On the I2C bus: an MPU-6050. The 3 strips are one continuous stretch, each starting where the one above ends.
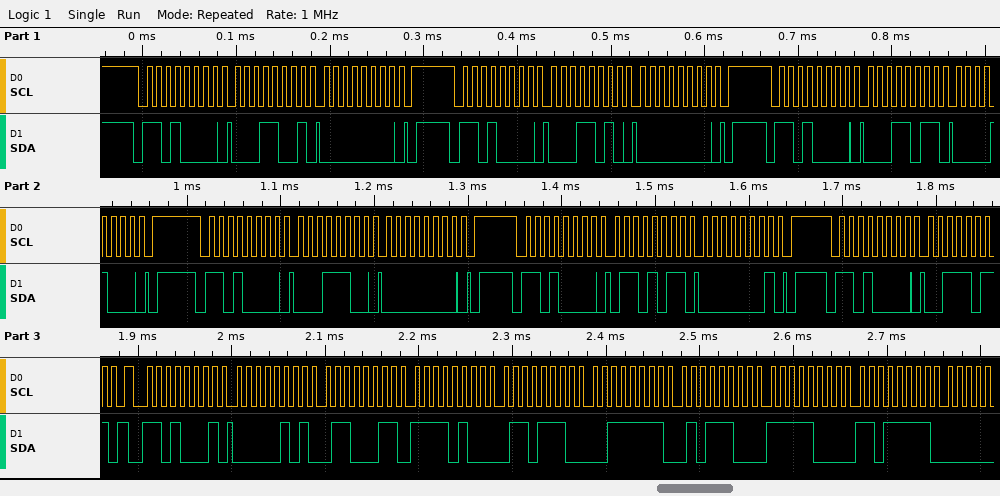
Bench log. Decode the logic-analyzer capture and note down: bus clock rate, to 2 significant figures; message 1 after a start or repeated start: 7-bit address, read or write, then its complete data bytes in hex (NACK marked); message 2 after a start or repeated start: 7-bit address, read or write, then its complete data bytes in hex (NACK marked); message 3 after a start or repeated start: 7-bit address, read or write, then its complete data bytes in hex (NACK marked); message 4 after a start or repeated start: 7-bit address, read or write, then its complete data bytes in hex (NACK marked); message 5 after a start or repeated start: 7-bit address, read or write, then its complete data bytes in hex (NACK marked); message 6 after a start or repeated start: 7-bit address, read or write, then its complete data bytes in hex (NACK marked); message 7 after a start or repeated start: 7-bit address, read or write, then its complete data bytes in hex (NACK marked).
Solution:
100 kHz
0x68 write: 19 00
0x68 write: 1A 00
0x68 write: 1B 08
0x68 write: 1C 00
0x68 write: 6B 01
0x68 write: 3B
0x68 read: 05 63 F4 6E 3F 5C F8 DF
